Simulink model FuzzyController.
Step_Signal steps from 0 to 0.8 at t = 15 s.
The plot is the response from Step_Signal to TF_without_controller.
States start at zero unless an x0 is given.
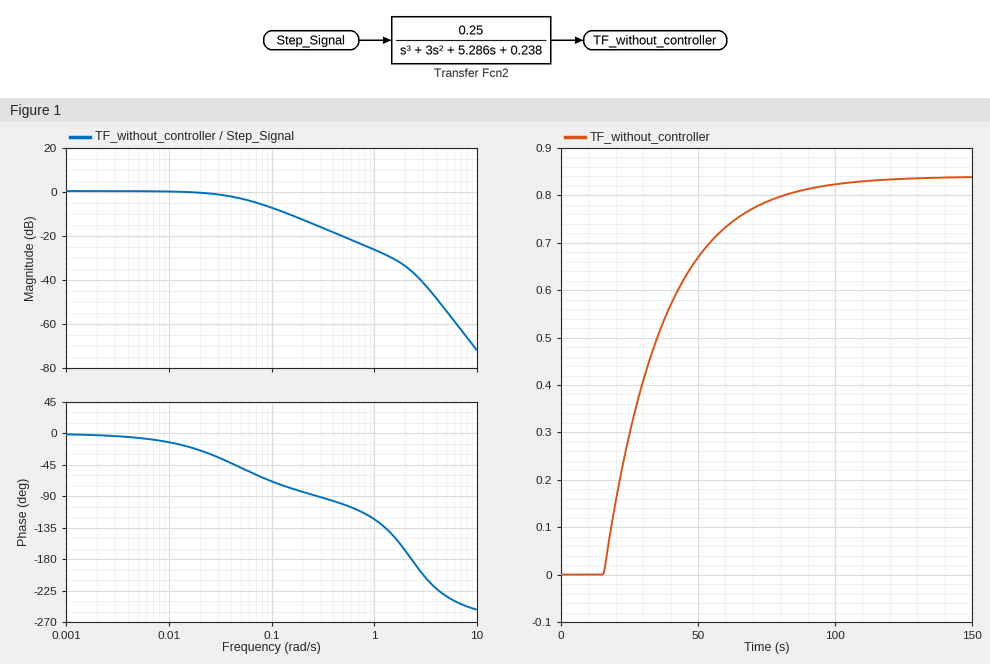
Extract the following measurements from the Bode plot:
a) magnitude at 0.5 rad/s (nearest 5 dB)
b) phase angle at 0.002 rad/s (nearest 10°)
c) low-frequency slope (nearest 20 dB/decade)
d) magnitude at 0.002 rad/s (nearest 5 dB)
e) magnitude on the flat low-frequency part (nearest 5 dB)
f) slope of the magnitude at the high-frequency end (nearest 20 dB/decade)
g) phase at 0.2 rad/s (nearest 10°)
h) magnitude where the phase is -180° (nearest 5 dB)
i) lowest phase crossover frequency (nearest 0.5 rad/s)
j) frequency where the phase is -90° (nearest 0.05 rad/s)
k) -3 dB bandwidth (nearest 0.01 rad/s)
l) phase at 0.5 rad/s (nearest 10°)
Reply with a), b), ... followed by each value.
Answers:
a) -20 dB
b) 0°
c) 0 dB/decade
d) 0 dB
e) 0 dB
f) -60 dB/decade
g) -80°
h) -35 dB
i) 2.5 rad/s
j) 0.30 rad/s
k) 0.05 rad/s
l) -100°
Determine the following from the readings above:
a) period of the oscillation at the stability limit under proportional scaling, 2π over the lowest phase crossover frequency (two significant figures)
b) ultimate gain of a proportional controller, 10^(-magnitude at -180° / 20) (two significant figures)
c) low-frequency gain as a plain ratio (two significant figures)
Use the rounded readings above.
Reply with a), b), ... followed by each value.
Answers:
a) 2.5 s
b) 56
c) 1.0
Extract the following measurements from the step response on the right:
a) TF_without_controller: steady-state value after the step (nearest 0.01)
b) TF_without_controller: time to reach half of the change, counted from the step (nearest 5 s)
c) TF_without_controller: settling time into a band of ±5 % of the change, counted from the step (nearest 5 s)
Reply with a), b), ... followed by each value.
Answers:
a) 0.84
b) 15 s
c) 65 s
